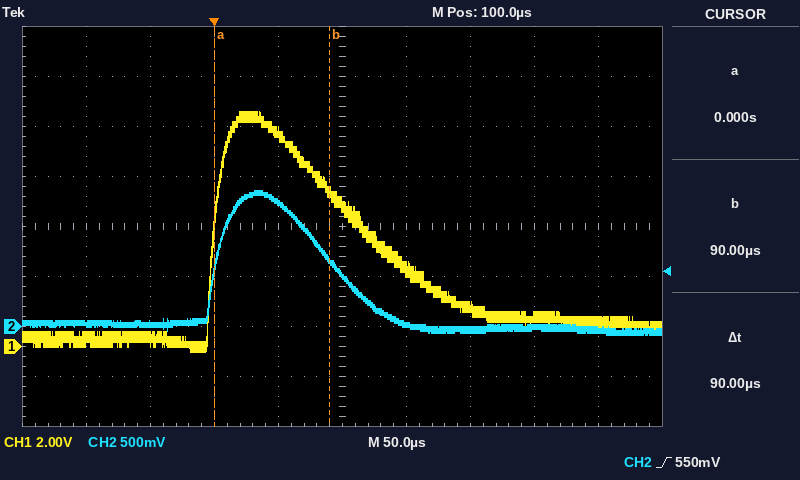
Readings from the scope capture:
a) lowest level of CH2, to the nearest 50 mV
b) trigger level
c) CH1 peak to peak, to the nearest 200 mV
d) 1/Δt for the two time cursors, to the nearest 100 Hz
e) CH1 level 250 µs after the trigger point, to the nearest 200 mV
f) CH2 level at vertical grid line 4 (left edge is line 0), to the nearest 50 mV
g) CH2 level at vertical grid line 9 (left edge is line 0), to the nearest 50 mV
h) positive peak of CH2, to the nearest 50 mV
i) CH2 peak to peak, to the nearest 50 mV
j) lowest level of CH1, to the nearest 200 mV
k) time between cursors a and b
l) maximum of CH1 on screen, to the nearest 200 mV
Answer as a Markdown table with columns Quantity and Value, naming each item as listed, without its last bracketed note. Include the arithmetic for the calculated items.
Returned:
| Quantity | Value |
|---|---|
| lowest level of CH2, to the nearest 50 mV | -100 mV |
| trigger level | 550 mV |
| CH1 peak to peak, to the nearest 200 mV | 9.4 V − (-200 mV) = 9.6 V |
| 1/Δt for the two time cursors, to the nearest 100 Hz | 1 / 90 µs ≈ 11.1 kHz |
| CH1 level 250 µs after the trigger point, to the nearest 200 mV | 1.2 V |
| CH2 level at vertical grid line 4 (left edge is line 0), to the nearest 50 mV | 1.25 V |
| CH2 level at vertical grid line 9 (left edge is line 0), to the nearest 50 mV | -50 mV |
| positive peak of CH2, to the nearest 50 mV | 1.35 V |
| CH2 peak to peak, to the nearest 50 mV | 1.35 V − (-100 mV) = 1.45 V |
| lowest level of CH1, to the nearest 200 mV | -200 mV |
| time between cursors a and b | 90 µs |
| maximum of CH1 on screen, to the nearest 200 mV | 9.4 V |
